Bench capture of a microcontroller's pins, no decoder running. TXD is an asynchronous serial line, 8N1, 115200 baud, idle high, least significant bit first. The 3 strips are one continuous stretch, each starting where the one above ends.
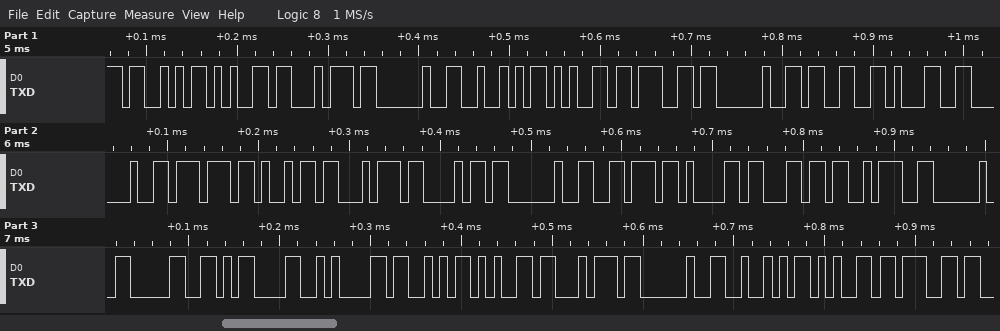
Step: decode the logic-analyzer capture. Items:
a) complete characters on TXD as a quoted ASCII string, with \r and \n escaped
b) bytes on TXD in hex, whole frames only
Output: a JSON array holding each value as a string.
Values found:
["\"Set Reg 31 with val: 0\\r\\nSet Reg\"", "53 65 74 20 52 65 67 20 33 31 20 77 69 74 68 20 76 61 6C 3A 20 30 0D 0A 53 65 74 20 52 65 67"]
